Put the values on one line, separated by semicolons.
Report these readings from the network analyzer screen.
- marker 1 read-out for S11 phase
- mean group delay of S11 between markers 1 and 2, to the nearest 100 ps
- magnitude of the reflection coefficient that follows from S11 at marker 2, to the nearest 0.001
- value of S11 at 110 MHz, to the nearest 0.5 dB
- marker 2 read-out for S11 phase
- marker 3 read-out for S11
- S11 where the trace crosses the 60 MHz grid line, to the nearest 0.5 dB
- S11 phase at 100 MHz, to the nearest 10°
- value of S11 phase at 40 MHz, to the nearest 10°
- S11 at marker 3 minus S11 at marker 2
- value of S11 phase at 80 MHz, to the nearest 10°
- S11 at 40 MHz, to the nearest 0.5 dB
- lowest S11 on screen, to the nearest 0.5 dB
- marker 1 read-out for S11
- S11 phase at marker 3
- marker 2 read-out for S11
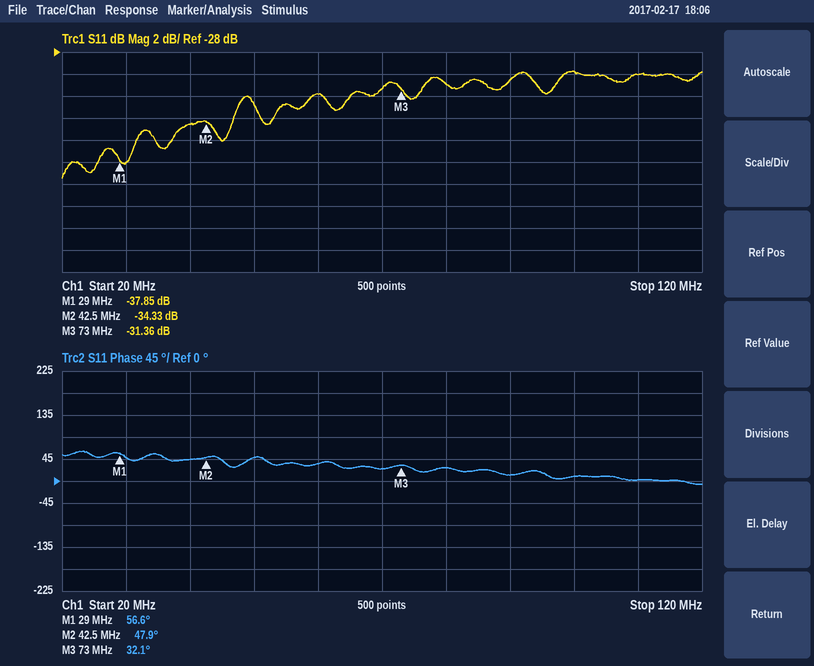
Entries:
56.6°; 1.8 ns; 0.019; -30.0 dB; 47.9°; -31.36 dB; -32.0 dB; 10°; 40°; 2.97 dB; 30°; -34.5 dB; -39.5 dB; -37.85 dB; 32.1°; -34.33 dB
